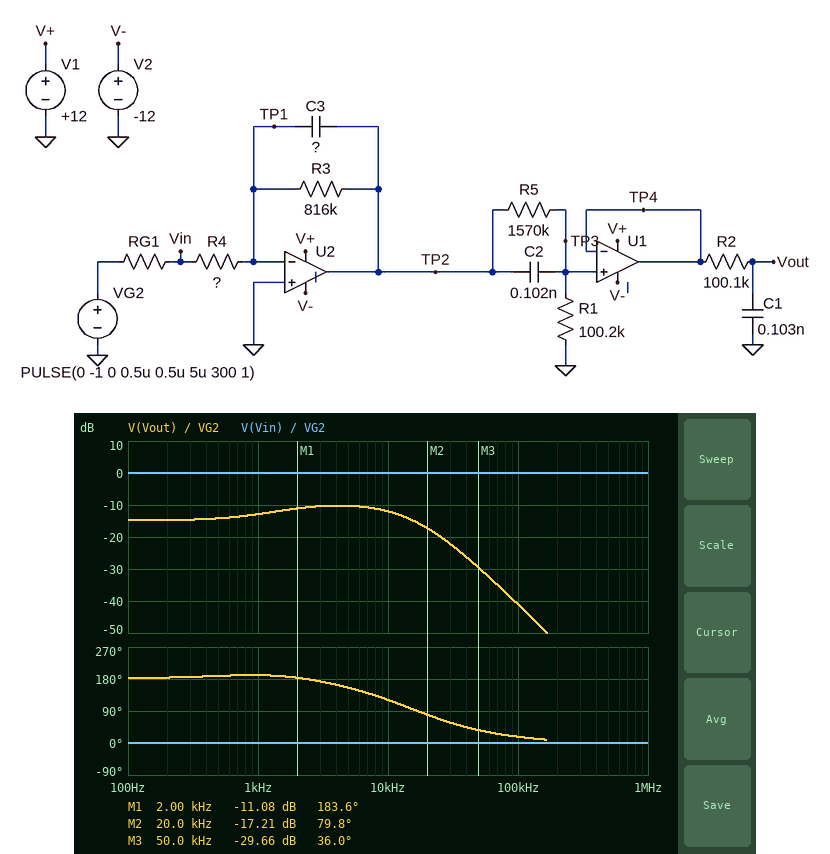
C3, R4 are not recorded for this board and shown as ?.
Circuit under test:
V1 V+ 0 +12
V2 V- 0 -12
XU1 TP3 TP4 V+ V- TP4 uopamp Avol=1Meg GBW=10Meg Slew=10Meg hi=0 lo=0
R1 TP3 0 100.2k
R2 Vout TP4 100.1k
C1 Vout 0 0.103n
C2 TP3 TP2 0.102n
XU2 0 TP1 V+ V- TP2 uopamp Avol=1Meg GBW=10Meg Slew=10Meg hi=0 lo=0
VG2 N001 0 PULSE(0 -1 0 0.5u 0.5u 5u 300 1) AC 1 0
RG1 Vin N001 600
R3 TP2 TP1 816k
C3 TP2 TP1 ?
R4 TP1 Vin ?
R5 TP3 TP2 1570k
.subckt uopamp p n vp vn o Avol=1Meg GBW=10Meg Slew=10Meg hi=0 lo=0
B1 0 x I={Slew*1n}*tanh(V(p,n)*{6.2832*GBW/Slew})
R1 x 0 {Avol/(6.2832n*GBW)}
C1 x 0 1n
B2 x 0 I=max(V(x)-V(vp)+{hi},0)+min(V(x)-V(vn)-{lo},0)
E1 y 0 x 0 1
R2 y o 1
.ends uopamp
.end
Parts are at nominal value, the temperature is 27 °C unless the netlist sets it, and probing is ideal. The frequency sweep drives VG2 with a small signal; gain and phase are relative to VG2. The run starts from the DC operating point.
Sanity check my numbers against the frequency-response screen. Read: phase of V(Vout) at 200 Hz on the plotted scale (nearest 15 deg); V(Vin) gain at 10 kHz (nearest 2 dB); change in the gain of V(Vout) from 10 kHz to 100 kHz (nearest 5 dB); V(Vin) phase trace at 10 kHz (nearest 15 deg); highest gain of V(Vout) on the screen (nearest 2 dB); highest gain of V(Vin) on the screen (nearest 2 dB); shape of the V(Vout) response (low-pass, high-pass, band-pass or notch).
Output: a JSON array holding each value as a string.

["180 deg", "0 dB", "-30 dB", "0 deg", "-10 dB", "0 dB", "low-pass"]
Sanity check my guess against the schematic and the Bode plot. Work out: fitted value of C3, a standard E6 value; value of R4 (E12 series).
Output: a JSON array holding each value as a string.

["100 pF", "270 kΩ"]
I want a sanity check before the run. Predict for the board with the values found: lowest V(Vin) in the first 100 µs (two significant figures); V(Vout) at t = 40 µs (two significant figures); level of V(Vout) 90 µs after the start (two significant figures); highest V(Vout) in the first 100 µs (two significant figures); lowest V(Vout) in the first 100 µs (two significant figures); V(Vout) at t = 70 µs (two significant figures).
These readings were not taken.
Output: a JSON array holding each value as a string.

["-1.0 V", "9.8 mV", "-4.9 mV", "68 mV", "-5.2 mV", "-5.0 mV"]
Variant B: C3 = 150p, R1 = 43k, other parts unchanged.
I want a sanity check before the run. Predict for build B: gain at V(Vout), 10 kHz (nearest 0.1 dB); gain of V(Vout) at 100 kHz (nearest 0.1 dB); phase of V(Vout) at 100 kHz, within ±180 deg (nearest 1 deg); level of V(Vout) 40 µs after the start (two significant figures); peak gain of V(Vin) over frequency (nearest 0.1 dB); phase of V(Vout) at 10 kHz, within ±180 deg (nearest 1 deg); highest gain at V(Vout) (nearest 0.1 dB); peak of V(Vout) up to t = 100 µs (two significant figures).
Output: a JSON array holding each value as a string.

["-21.4 dB", "-45.0 dB", "28 deg", "1.8 mV", "0 dB", "134 deg", "-20.0 dB", "29 mV"]
